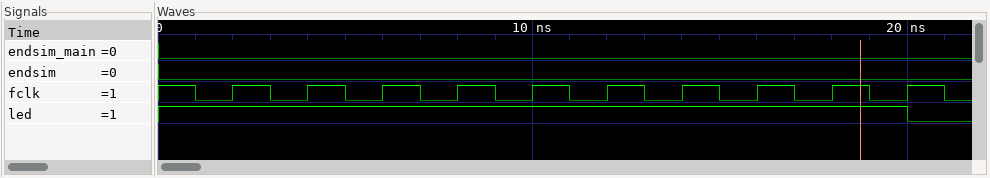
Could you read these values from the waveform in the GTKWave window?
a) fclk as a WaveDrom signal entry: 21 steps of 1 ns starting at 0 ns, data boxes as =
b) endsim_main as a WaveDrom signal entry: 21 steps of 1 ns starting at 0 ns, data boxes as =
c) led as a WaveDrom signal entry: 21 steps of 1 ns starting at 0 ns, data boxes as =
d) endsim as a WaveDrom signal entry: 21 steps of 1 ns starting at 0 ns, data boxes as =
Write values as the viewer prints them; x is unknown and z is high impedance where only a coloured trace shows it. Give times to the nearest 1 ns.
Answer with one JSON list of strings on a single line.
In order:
["{name: 'fclk', wave: '101010101010101010101'}", "{name: 'endsim_main', wave: '0....................'}", "{name: 'led', wave: '1...................0'}", "{name: 'endsim', wave: '0....................'}"]
